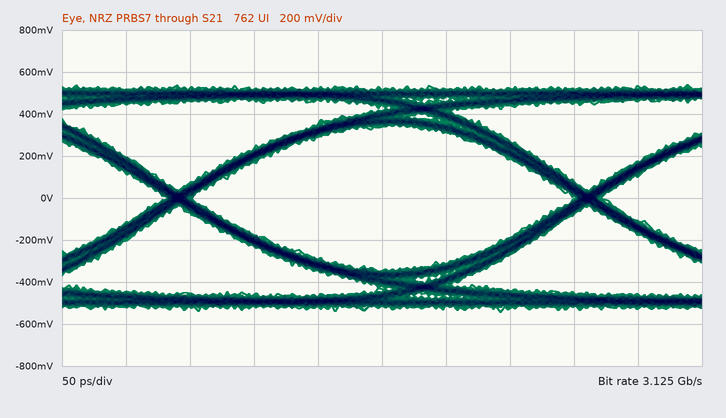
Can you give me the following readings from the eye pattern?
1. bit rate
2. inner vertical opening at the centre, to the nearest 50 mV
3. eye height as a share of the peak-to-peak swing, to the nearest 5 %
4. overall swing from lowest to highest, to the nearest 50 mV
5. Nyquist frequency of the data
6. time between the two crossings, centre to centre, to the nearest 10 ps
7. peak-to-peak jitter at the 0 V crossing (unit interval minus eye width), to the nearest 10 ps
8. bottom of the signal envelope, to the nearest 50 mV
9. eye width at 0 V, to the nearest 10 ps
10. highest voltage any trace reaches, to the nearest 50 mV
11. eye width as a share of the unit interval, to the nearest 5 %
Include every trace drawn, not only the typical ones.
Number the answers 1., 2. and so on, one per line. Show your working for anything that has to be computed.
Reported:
1. 3.125 Gb/s
2. 700 mV
3. 700 mV / 1.10 V ≈ 63.6 %, so 65 % to the nearest 5 %
4. 1.10 V
5. 1.5625 GHz
6. 320 ps
7. 20 ps
8. -550 mV
9. 300 ps
10. 550 mV
11. 300 ps / 320 ps ≈ 93.8 %, so 95 % to the nearest 5 %
